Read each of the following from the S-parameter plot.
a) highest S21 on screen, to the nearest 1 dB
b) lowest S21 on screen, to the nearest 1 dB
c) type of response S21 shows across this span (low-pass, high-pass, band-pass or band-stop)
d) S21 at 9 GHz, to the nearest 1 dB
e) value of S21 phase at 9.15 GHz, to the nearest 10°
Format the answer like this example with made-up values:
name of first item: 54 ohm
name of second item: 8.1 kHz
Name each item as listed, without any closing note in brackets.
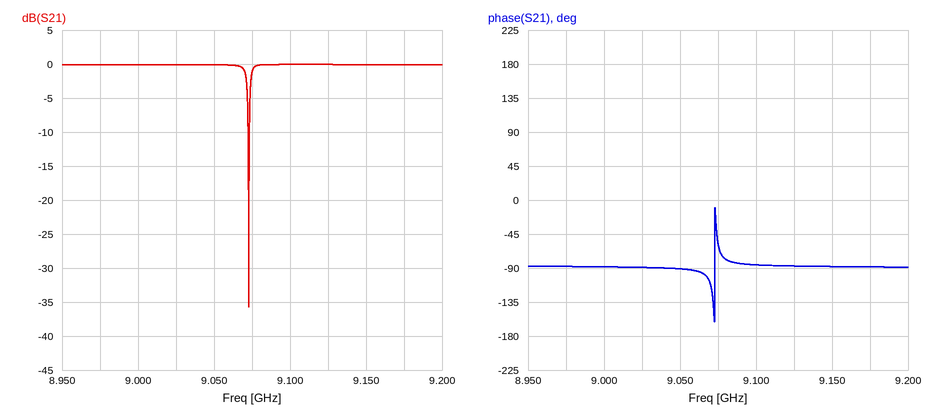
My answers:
highest S21 on screen, to the nearest 1 dB: 0 dB
lowest S21 on screen, to the nearest 1 dB: -36 dB
type of response S21 shows across this span: band-stop
S21 at 9 GHz, to the nearest 1 dB: 0 dB
value of S21 phase at 9.15 GHz, to the nearest 10°: -90°
